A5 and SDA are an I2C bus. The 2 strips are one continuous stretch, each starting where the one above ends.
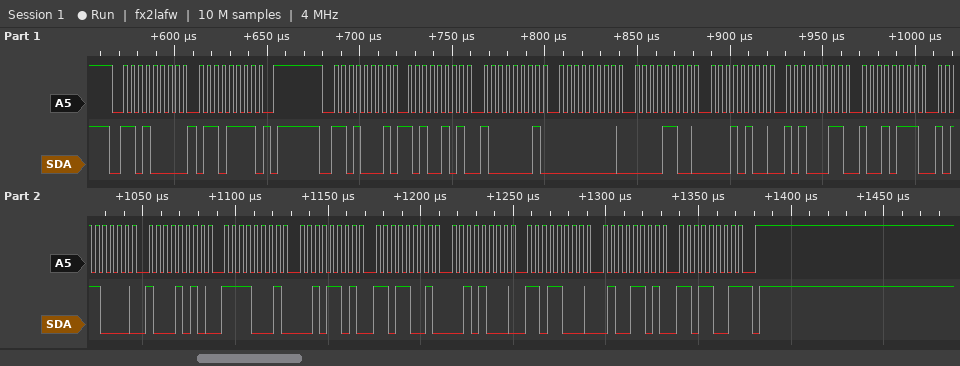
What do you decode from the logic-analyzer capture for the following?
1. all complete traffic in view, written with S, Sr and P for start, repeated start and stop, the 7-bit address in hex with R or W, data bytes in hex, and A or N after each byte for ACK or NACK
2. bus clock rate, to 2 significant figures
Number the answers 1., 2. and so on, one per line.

1. S 68W A 6F A P S 68R A A5 A 81 A 00 A 0C A 14 A A3 A 97 A B0 A 8A A F1 A 2D A D9 A 28 A D8 A 4D A D9 N P
2. 250 kHz
